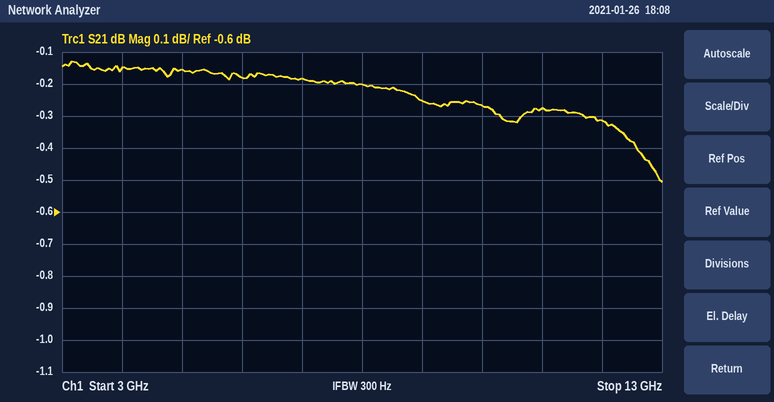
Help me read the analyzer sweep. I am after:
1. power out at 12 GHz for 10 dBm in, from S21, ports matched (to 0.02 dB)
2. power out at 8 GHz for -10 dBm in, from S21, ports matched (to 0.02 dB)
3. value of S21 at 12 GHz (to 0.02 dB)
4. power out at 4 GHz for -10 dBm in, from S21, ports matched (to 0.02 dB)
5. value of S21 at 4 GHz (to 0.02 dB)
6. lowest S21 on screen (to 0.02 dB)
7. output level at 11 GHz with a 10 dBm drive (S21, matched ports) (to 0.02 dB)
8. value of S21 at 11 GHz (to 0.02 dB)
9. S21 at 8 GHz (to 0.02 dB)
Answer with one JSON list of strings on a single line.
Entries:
["9.68 dBm", "-10.20 dBm", "-0.32 dB", "-10.16 dBm", "-0.16 dB", "-0.50 dB", "9.72 dBm", "-0.28 dB", "-0.20 dB"]
